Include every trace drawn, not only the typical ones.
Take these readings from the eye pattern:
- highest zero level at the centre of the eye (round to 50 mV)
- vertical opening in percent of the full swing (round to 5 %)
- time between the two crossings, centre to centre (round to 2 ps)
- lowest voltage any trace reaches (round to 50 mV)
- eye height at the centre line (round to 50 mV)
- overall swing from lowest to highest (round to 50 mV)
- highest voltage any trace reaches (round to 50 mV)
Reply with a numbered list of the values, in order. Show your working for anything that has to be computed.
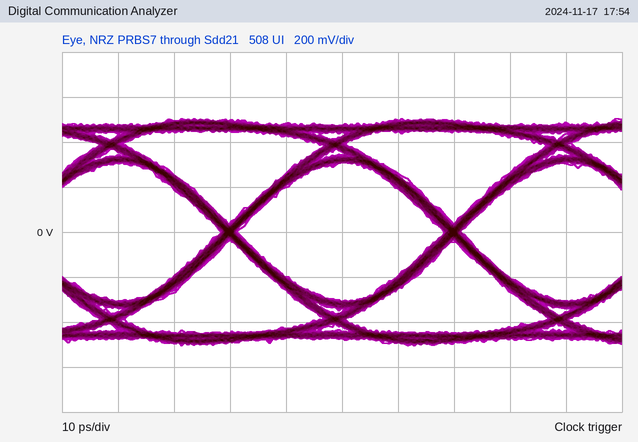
1. -300 mV
2. 600 mV / 1.00 V ≈ 60 %
3. 40 ps
4. -500 mV
5. 600 mV
6. 1.00 V
7. 500 mV
